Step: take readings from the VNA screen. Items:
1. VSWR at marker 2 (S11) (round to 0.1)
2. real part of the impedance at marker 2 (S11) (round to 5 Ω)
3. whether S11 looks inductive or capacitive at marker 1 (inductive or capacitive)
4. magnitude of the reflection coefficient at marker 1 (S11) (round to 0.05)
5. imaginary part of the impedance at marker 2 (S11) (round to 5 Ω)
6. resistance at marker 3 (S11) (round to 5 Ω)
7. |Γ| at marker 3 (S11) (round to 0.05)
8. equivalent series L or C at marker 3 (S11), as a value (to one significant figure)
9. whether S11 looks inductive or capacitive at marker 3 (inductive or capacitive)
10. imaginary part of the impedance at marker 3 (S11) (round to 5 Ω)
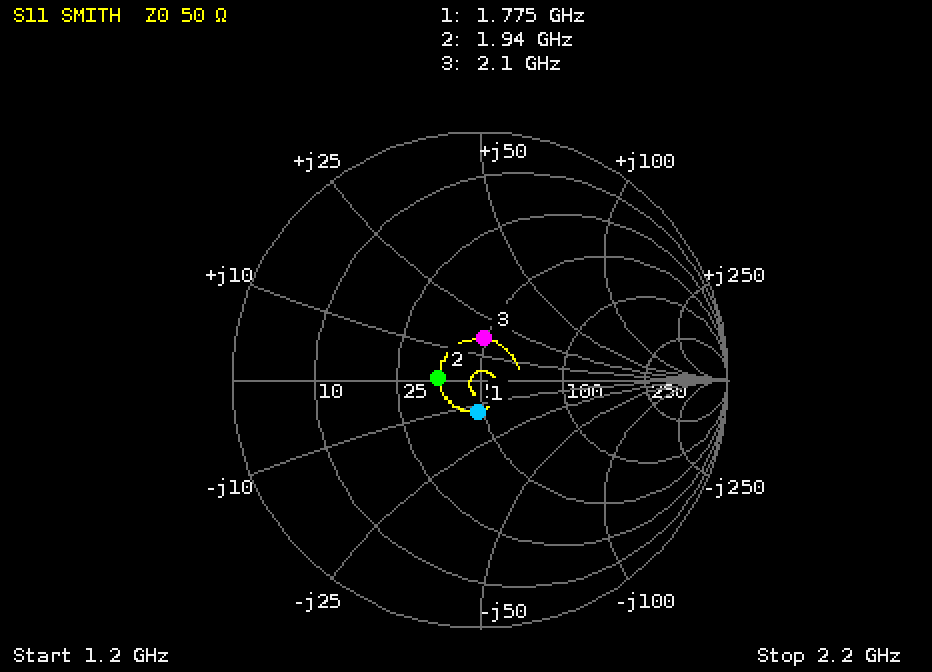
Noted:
1.4
35 Ω
capacitive
0.15
0 Ω
50 Ω
0.15
1 nH
inductive
+15 Ω
